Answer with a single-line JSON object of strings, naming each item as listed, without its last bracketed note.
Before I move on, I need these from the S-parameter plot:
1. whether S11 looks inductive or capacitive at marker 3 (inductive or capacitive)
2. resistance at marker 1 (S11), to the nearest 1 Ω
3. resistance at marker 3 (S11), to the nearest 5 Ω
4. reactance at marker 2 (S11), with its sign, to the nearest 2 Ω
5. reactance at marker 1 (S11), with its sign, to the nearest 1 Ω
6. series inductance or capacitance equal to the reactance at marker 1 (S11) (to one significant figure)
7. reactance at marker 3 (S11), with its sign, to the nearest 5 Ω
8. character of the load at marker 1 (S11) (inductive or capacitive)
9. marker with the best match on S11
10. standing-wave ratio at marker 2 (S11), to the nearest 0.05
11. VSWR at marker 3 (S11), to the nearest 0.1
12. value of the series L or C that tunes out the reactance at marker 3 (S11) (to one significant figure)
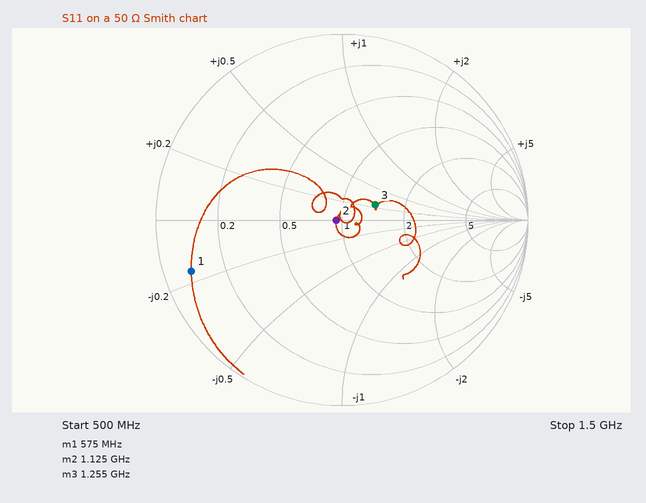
{"whether S11 looks inductive or capacitive at marker 3": "inductive", "resistance at marker 1 (S11), to the nearest 1 Ω": "4 Ω", "resistance at marker 3 (S11), to the nearest 5 Ω": "70 Ω", "reactance at marker 2 (S11), with its sign, to the nearest 2 Ω": "0 Ω", "reactance at marker 1 (S11), with its sign, to the nearest 1 Ω": "-8 Ω", "series inductance or capacitance equal to the reactance at marker 1 (S11)": "30 pF", "reactance at marker 3 (S11), with its sign, to the nearest 5 Ω": "+10 Ω", "character of the load at marker 1 (S11)": "capacitive", "marker with the best match on S11": "marker 2", "standing-wave ratio at marker 2 (S11), to the nearest 0.05": "1.05", "VSWR at marker 3 (S11), to the nearest 0.1": "1.5", "value of the series L or C that tunes out the reactance at marker 3 (S11)": "10 pF"}
